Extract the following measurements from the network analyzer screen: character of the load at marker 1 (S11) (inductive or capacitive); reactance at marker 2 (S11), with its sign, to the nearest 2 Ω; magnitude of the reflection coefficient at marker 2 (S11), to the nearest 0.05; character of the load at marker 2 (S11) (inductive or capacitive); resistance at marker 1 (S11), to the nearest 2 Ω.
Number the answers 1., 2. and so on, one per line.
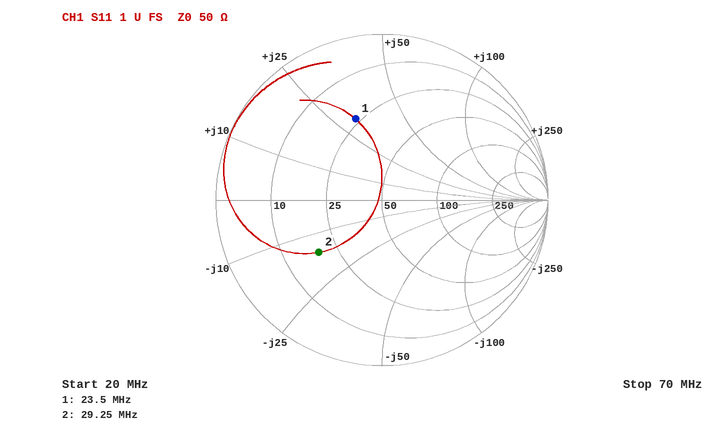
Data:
1. inductive
2. -16 Ω
3. 0.50
4. capacitive
5. 24 Ω
